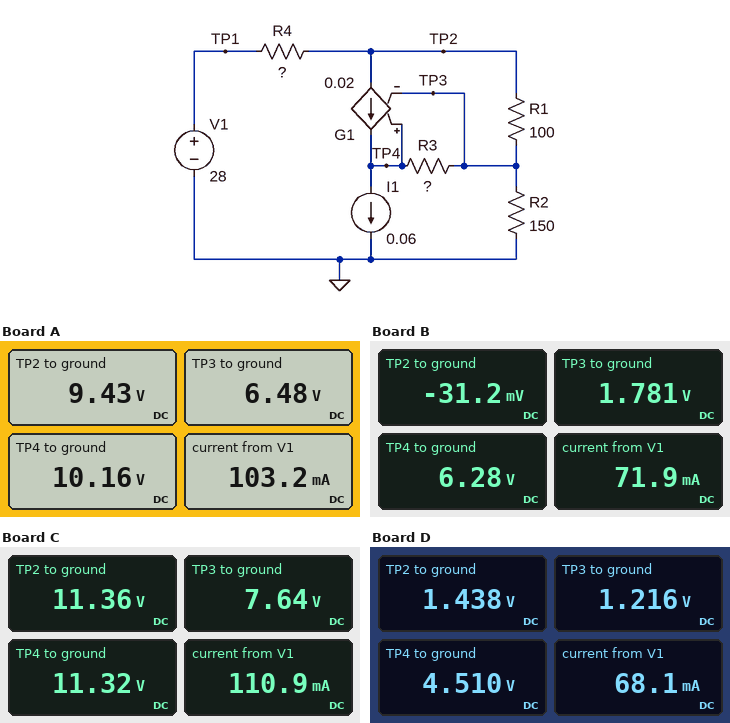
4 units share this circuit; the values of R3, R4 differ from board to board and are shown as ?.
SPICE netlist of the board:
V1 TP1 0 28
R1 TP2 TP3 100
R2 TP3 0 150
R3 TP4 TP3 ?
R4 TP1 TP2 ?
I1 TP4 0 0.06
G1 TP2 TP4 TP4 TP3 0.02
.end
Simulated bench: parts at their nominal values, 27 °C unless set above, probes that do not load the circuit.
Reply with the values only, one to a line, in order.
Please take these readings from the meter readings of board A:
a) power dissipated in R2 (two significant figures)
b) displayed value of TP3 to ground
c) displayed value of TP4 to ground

280 mW
6.48 V
10.16 V
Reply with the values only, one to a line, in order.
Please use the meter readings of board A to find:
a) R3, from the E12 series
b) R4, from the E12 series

270 Ω
180 Ω
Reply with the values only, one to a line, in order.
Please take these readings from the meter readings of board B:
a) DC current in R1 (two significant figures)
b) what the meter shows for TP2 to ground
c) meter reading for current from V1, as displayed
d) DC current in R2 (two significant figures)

18 mA
-31.2 mV
71.9 mA
12 mA
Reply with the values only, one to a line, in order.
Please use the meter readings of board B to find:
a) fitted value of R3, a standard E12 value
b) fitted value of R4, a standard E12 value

150 Ω
390 Ω
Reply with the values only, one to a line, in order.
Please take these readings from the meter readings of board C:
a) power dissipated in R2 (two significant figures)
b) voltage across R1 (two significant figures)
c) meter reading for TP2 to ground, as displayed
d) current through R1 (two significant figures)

390 mW
3.7 V
11.36 V
37 mA
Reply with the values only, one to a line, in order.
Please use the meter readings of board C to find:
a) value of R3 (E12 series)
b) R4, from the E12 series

270 Ω
150 Ω
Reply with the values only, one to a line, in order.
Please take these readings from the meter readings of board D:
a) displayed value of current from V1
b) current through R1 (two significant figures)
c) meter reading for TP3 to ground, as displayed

68.1 mA
2.2 mA
1.216 V
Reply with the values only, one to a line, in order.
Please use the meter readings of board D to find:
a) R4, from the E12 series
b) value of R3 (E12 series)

390 Ω
560 Ω
